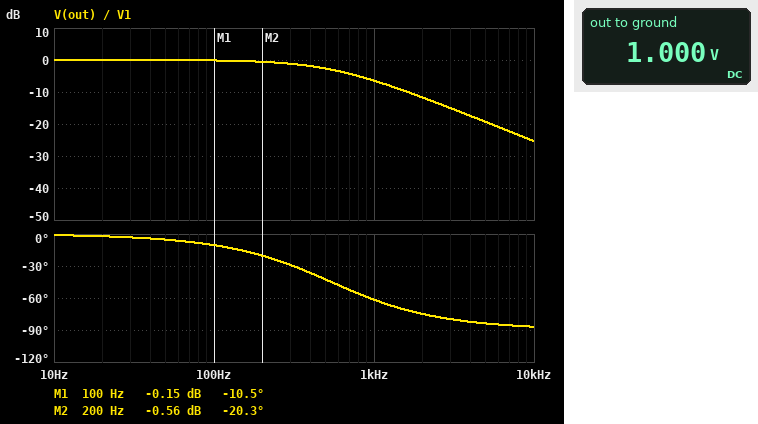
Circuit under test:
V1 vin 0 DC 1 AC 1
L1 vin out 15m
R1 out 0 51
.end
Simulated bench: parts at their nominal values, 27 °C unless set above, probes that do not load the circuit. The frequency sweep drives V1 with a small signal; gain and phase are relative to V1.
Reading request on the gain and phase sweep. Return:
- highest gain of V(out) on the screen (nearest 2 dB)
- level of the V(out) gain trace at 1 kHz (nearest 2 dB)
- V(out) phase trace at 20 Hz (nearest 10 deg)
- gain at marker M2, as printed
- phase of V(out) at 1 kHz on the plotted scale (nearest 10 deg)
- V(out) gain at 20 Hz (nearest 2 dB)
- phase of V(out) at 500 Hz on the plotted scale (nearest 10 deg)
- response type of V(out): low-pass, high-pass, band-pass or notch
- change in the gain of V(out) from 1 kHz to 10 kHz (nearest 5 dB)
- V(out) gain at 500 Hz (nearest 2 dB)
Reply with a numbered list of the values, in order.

1. 0 dB
2. -6 dB
3. 0 deg
4. -0.56 dB
5. -60 deg
6. 0 dB
7. -40 deg
8. low-pass
9. -20 dB
10. -2 dB
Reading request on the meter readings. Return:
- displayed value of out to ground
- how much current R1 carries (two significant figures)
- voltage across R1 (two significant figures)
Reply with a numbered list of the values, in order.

1. 1.000 V
2. 20 mA
3. 1.0 V
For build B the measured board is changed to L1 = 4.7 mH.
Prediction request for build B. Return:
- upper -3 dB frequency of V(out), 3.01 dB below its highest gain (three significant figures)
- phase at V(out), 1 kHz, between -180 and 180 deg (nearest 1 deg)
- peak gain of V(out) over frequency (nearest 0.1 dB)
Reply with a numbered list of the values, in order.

1. 1.73 kHz
2. -30 deg
3. 0 dB
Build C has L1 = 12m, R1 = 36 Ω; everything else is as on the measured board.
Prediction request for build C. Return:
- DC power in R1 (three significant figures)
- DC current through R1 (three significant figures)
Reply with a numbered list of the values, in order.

1. 27.8 mW
2. 27.8 mA
